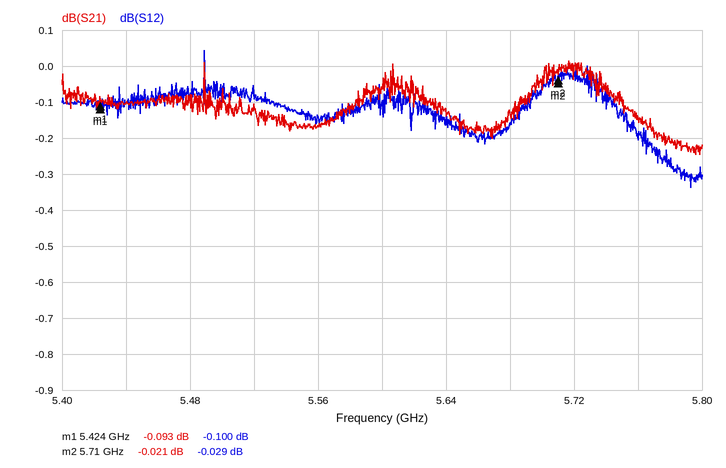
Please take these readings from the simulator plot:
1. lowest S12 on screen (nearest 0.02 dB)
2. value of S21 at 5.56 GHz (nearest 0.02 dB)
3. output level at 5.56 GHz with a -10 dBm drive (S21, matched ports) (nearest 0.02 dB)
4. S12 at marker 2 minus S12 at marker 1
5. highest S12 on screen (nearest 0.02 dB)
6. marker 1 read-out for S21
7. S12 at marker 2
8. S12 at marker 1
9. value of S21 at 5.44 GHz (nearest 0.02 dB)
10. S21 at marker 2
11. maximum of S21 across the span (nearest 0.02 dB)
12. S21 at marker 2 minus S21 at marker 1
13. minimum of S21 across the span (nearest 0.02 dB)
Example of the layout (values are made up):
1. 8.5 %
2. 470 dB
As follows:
1. -0.34 dB
2. -0.16 dB
3. -10.16 dBm
4. 0.071 dB
5. 0.04 dB
6. -0.093 dB
7. -0.029 dB
8. -0.100 dB
9. -0.10 dB
10. -0.021 dB
11. 0.02 dB
12. 0.072 dB
13. -0.24 dB
